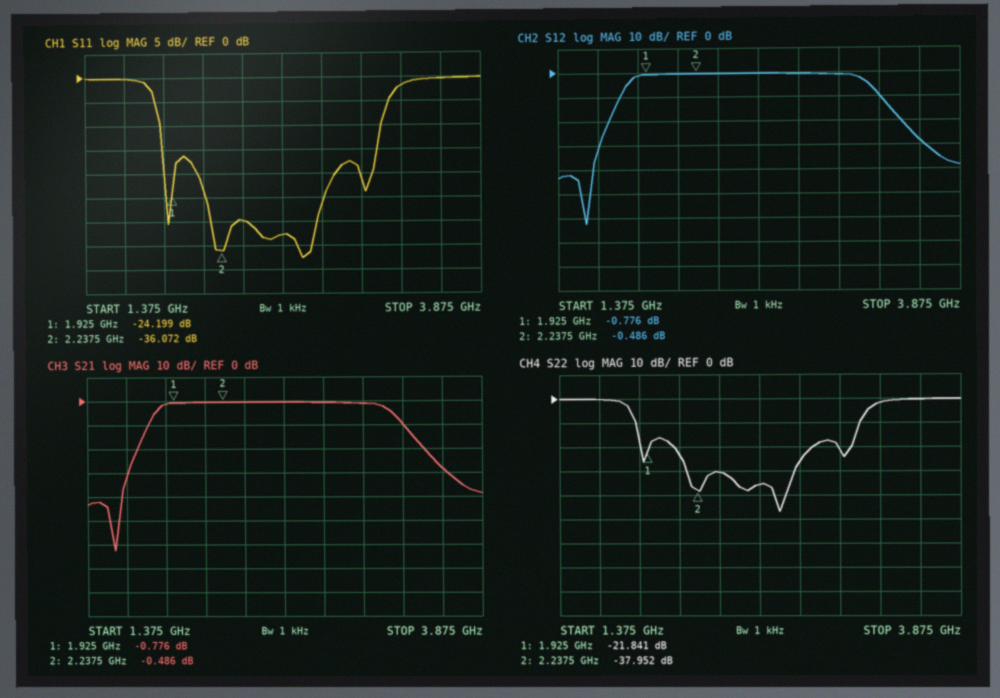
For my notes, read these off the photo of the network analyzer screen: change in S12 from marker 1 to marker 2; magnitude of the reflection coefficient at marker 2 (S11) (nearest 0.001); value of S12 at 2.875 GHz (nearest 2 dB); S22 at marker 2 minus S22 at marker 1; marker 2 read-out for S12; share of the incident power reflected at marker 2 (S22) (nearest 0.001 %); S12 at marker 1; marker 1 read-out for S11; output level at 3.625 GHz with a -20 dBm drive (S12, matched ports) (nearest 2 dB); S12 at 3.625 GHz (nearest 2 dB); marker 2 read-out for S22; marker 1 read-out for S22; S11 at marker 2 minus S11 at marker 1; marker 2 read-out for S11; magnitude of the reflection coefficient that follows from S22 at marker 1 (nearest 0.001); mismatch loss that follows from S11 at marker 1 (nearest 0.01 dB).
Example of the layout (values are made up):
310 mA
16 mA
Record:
0.290 dB
0.016
0 dB
-16.111 dB
-0.486 dB
0.016 %
-0.776 dB
-24.199 dB
-48 dBm
-28 dB
-37.952 dB
-21.841 dB
-11.873 dB
-36.072 dB
0.081
0.02 dB
